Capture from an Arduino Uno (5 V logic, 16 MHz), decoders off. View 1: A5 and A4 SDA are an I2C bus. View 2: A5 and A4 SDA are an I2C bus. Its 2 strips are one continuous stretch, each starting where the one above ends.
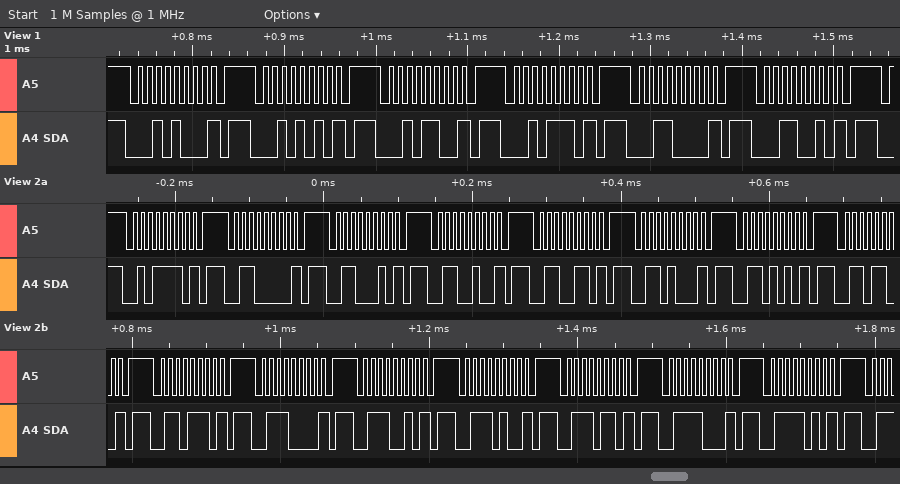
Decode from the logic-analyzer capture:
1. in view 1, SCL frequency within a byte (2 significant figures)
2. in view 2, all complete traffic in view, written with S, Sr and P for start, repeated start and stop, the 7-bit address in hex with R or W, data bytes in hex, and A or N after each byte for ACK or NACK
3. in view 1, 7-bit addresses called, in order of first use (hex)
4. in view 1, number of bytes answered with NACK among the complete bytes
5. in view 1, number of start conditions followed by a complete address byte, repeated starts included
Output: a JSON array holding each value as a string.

["100 kHz", "S 2FW N P S 30W N P S 31W N P S 32W N P S 33W N P S 34W N P S 35W N P S 36W N P S 37W N P S 38W N P S 39W N P S 3AW N P S 3BW N P S 3CW N P S 3DW N P", "0x14 0x15 0x16 0x17 0x18 0x19", "6", "6"]
